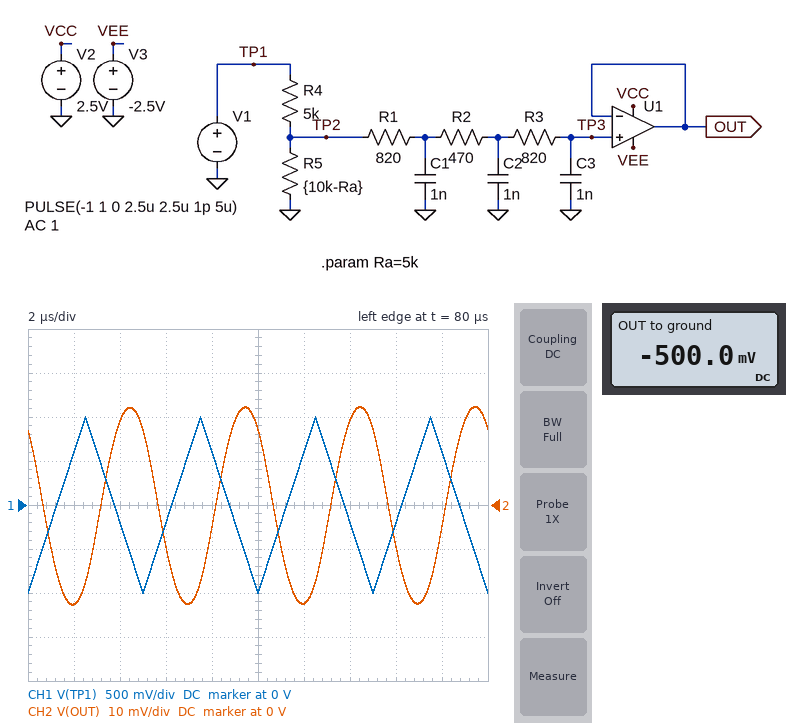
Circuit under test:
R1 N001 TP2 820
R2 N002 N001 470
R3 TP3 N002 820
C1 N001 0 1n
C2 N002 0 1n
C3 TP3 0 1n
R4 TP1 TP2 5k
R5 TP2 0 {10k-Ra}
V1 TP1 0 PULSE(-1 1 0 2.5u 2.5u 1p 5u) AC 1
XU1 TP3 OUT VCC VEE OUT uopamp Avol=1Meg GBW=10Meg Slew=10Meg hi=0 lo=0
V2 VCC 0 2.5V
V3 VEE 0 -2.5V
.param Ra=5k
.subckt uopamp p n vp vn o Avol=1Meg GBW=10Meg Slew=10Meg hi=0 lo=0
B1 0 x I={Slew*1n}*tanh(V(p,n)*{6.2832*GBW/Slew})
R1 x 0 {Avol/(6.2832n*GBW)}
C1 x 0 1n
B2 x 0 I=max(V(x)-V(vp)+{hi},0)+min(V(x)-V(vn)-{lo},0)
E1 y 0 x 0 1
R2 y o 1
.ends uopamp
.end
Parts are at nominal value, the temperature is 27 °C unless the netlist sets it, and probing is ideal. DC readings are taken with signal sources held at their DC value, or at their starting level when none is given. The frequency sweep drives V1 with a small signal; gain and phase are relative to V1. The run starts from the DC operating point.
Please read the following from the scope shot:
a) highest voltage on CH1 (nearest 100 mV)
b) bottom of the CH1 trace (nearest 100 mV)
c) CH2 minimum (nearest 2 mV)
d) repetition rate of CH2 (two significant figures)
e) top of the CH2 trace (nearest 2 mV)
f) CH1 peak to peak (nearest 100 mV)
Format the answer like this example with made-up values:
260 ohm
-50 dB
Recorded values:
1.0 V
-1.0 V
-22 mV
200 kHz
22 mV
2.0 V
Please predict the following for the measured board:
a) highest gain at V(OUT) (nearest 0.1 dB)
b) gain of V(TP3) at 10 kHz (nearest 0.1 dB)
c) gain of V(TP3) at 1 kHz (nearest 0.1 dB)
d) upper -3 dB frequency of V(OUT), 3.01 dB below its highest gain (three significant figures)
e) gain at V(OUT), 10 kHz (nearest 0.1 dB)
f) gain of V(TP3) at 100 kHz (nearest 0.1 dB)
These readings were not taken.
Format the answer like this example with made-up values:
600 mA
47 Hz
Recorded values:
-6.0 dB
-7.7 dB
-6.0 dB
14.5 kHz
-7.7 dB
-23.5 dB
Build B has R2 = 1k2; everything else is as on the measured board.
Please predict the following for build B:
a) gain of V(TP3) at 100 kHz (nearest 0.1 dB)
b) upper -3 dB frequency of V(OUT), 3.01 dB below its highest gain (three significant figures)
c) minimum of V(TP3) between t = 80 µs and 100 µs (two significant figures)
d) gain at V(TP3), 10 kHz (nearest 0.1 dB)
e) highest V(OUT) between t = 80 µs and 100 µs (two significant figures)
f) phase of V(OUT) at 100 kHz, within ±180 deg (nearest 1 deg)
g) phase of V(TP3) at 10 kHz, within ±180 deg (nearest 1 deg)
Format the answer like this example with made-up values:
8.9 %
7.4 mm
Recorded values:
-24.9 dB
13.2 kHz
-17 mV
-8.0 dB
17 mV
-123 deg
-41 deg
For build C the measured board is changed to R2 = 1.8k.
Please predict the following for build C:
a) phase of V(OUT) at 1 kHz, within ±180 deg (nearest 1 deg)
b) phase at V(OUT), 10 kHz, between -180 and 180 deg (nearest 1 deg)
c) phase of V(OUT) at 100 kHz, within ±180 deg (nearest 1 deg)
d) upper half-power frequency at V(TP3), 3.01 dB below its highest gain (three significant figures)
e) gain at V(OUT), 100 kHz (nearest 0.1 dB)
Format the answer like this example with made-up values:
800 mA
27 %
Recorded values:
-5 deg
-44 deg
-130 deg
12.2 kHz
-26.1 dB
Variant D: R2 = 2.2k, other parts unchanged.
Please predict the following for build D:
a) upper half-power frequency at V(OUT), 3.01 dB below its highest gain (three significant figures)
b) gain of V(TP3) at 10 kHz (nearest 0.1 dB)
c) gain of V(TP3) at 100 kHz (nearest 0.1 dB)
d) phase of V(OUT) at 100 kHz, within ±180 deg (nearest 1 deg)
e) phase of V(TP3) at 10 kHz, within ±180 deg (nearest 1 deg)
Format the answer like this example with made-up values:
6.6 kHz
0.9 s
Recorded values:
11.6 kHz
-8.4 dB
-26.9 dB
-134 deg
-46 deg
